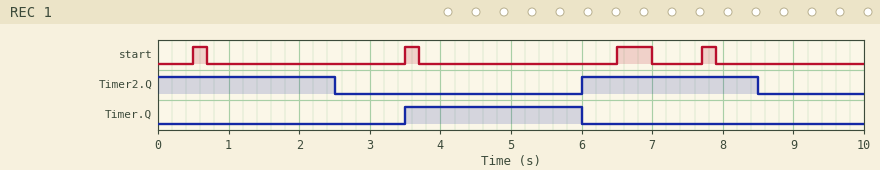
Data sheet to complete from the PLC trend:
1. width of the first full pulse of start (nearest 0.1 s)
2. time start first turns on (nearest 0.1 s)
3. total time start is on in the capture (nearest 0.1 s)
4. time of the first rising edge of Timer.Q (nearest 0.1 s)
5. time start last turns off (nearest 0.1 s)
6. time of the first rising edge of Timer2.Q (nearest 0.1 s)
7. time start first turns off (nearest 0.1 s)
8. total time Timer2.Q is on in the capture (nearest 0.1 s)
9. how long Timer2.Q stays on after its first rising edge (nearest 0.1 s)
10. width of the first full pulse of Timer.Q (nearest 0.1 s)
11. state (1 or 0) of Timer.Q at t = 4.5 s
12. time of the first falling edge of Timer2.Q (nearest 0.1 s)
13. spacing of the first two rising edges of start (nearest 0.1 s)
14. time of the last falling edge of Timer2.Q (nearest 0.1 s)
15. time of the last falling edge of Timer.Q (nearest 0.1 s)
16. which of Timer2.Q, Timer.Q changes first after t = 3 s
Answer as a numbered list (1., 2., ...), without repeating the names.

1. 0.2 s
2. 0.5 s
3. 1.1 s
4. 3.5 s
5. 7.9 s
6. 6.0 s
7. 0.7 s
8. 5.0 s
9. 2.5 s
10. 2.5 s
11. 1
12. 2.5 s
13. 3.0 s
14. 8.5 s
15. 6.0 s
16. Timer.Q
